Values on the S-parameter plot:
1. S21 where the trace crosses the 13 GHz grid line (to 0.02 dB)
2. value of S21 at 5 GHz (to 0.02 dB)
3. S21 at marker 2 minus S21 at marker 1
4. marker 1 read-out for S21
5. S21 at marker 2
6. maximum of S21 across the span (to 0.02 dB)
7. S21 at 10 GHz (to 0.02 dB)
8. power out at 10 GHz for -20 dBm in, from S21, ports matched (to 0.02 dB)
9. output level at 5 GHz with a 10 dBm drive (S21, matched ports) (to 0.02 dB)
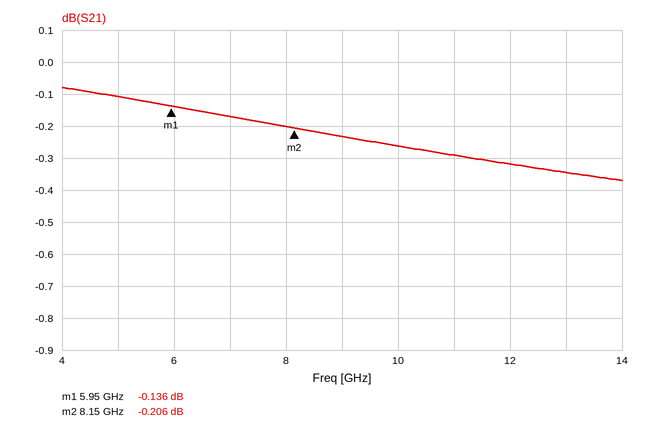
-0.34 dB
-0.10 dB
-0.070 dB
-0.136 dB
-0.206 dB
-0.08 dB
-0.26 dB
-20.26 dBm
9.90 dBm
